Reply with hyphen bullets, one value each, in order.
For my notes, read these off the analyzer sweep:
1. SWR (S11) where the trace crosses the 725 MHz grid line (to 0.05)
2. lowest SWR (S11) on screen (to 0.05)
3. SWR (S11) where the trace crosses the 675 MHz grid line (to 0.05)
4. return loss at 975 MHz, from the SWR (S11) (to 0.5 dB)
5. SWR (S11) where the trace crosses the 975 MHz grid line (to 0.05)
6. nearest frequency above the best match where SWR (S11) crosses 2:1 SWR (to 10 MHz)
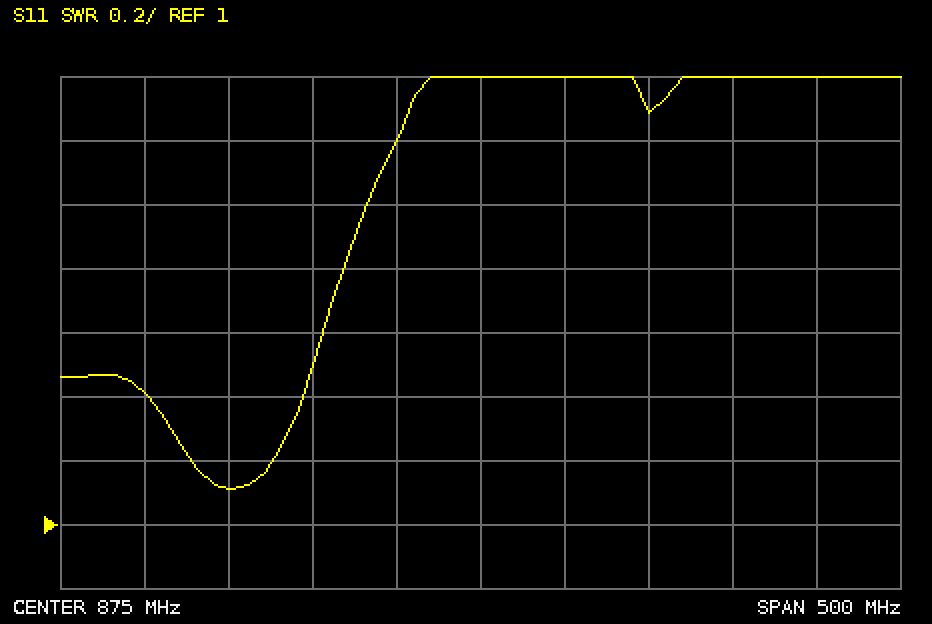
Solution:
- 1.10
- 1.10
- 1.40
- 8.0 dB
- 2.30
- 810 MHz
